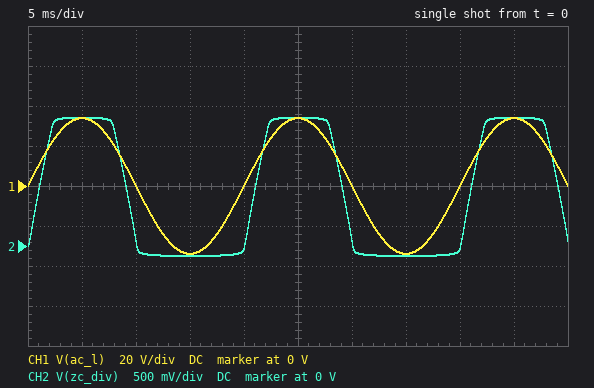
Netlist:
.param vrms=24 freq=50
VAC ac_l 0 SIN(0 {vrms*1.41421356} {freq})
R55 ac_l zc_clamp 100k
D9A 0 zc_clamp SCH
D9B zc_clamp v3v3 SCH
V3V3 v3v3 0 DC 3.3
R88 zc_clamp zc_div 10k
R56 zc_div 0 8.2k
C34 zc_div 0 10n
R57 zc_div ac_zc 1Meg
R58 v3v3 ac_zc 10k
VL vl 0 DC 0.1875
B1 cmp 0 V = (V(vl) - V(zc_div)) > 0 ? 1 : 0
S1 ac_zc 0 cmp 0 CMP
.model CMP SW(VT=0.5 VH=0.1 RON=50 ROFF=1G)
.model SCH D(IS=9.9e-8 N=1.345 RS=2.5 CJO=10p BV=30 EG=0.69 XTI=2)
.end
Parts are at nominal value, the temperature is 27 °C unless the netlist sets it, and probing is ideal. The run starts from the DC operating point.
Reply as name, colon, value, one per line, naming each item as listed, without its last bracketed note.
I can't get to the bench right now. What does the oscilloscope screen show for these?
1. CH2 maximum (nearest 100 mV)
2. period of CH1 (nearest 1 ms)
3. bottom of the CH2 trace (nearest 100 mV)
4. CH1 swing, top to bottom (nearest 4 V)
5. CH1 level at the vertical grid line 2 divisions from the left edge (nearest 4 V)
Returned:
CH2 maximum: 1.6 V
period of CH1: 20 ms
bottom of the CH2 trace: -100 mV
CH1 swing, top to bottom: 68 V
CH1 level at the vertical grid line 2 divisions from the left edge: 0 V
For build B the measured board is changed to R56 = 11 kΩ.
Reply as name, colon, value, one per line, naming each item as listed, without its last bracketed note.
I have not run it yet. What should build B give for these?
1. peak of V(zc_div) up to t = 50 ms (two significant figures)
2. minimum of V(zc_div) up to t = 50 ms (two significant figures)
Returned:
peak of V(zc_div) up to t = 50 ms: 1.9 V
minimum of V(zc_div) up to t = 50 ms: -150 mV
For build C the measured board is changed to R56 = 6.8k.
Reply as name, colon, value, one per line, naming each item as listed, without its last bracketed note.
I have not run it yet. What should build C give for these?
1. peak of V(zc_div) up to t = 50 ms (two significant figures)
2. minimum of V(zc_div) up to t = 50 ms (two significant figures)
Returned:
peak of V(zc_div) up to t = 50 ms: 1.4 V
minimum of V(zc_div) up to t = 50 ms: -110 mV
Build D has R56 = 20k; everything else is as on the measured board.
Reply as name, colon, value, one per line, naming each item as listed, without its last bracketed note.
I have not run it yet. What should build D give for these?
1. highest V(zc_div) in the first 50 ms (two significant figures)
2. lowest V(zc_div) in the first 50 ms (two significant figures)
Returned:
highest V(zc_div) in the first 50 ms: 2.4 V
lowest V(zc_div) in the first 50 ms: -190 mV
